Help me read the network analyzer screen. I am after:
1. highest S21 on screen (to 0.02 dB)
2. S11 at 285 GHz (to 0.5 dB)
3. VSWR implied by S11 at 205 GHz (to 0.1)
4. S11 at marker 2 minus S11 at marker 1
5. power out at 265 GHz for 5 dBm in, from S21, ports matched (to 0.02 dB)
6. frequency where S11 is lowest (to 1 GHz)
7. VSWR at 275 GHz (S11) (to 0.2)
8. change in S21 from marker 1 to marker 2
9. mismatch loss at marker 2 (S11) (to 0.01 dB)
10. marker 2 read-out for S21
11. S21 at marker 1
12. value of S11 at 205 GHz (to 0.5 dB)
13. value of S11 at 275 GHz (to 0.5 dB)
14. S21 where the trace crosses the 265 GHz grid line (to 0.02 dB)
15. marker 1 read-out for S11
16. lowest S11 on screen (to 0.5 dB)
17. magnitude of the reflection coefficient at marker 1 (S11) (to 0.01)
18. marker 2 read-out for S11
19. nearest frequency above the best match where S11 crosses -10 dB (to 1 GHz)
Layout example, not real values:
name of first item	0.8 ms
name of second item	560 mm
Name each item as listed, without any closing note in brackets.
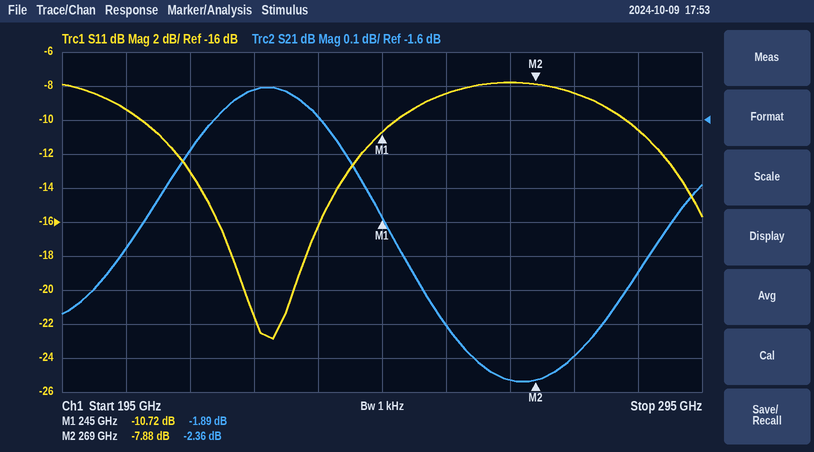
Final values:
highest S21 on screen	-1.50 dB
S11 at 285 GHz	-10.5 dB
VSWR implied by S11 at 205 GHz	2.0
S11 at marker 2 minus S11 at marker 1	2.84 dB
power out at 265 GHz for 5 dBm in, from S21, ports matched	2.64 dBm
frequency where S11 is lowest	228 GHz
VSWR at 275 GHz (S11)	2.2
change in S21 from marker 1 to marker 2	-0.47 dB
mismatch loss at marker 2 (S11)	0.77 dB
marker 2 read-out for S21	-2.36 dB
S21 at marker 1	-1.89 dB
value of S11 at 205 GHz	-9.5 dB
value of S11 at 275 GHz	-8.5 dB
S21 where the trace crosses the 265 GHz grid line	-2.36 dB
marker 1 read-out for S11	-10.72 dB
lowest S11 on screen	-23.0 dB
magnitude of the reflection coefficient at marker 1 (S11)	0.29
marker 2 read-out for S11	-7.88 dB
nearest frequency above the best match where S11 crosses -10 dB	247 GHz
